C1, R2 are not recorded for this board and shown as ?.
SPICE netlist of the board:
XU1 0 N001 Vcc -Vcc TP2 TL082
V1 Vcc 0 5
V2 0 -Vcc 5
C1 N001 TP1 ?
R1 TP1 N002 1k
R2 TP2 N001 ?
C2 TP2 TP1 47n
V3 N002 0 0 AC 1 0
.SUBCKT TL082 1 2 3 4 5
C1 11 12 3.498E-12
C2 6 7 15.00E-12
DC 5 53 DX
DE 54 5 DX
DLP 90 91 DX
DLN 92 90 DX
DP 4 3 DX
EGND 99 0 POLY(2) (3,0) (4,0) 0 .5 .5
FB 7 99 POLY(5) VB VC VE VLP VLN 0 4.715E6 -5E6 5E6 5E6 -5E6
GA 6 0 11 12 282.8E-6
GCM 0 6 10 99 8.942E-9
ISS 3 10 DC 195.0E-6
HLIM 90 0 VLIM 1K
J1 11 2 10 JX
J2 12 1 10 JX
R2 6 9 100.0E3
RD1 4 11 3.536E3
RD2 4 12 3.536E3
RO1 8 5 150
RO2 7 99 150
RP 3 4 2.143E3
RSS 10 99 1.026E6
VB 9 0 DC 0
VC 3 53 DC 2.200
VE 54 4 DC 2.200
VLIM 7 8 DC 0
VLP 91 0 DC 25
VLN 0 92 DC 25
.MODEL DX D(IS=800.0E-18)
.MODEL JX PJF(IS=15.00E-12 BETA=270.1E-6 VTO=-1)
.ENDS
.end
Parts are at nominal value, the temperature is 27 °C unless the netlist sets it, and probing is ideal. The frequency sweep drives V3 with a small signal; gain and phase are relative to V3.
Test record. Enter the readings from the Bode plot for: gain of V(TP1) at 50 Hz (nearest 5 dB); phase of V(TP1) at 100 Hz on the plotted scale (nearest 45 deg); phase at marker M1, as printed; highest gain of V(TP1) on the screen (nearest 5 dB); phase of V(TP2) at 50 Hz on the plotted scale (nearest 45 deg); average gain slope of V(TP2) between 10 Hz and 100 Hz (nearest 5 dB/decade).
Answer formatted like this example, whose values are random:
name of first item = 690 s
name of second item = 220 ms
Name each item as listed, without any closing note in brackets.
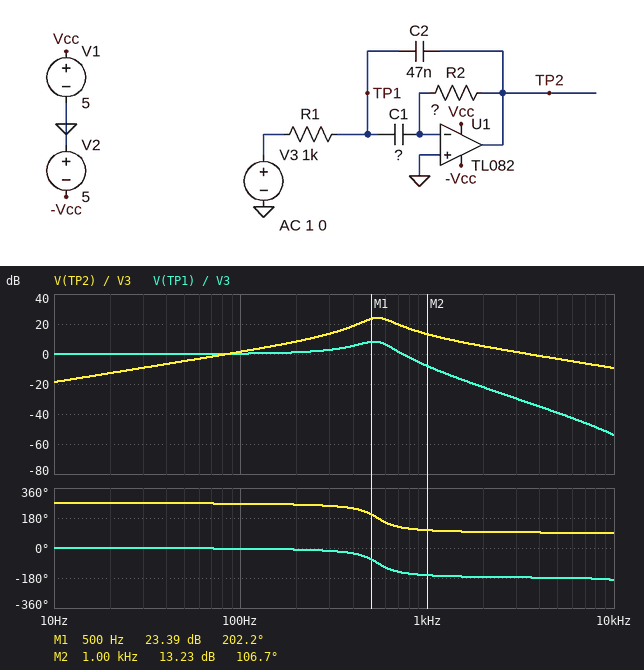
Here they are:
gain of V(TP1) at 50 Hz = 0 dB
phase of V(TP1) at 100 Hz on the plotted scale = 0 deg
phase at marker M1, as printed = 202.2 deg
highest gain of V(TP1) on the screen = 10 dB
phase of V(TP2) at 50 Hz on the plotted scale = 270 deg
average gain slope of V(TP2) between 10 Hz and 100 Hz = 20 dB/decade
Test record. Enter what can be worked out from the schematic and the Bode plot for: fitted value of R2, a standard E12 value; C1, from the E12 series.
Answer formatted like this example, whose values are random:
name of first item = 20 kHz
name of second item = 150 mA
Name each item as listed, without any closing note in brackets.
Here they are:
fitted value of R2, a standard E12 value = 27 kΩ
C1, from the E12 series = 68 nF
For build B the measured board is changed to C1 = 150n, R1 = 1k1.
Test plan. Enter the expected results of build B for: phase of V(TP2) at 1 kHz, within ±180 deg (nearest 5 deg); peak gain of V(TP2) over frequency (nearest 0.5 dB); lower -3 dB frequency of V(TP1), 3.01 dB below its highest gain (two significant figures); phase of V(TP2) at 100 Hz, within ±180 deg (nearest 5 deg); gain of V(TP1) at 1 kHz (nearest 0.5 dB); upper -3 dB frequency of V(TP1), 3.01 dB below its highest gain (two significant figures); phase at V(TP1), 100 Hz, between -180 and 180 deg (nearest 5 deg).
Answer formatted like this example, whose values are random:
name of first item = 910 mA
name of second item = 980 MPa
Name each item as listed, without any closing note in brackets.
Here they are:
phase of V(TP2) at 1 kHz, within ±180 deg = 100 deg
peak gain of V(TP2) over frequency = 25.5 dB
lower -3 dB frequency of V(TP1), 3.01 dB below its highest gain = 230 Hz
phase of V(TP2) at 100 Hz, within ±180 deg = -100 deg
gain of V(TP1) at 1 kHz = -17.5 dB
upper -3 dB frequency of V(TP1), 3.01 dB below its highest gain = 400 Hz
phase at V(TP1), 100 Hz, between -180 and 180 deg = -10 deg
